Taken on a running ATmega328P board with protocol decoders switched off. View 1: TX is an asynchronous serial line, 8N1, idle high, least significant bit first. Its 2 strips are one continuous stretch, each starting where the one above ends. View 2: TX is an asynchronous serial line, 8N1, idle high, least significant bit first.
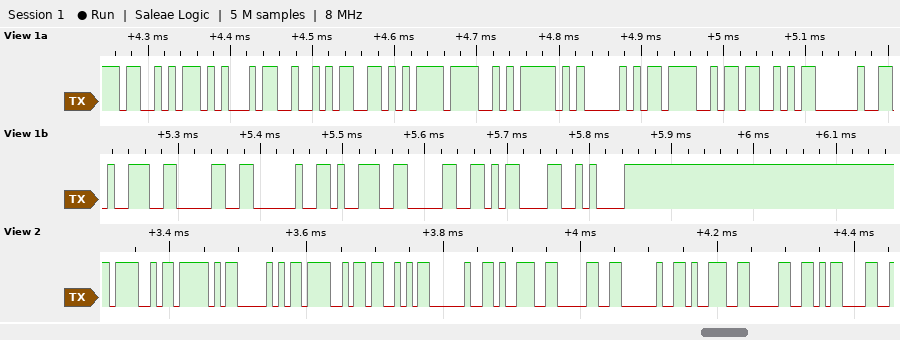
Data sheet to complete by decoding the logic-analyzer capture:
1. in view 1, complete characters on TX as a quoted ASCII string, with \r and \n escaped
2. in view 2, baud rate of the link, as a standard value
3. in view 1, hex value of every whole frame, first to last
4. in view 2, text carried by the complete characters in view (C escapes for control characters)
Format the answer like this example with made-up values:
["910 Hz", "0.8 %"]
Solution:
["\"SERVO_POS 90 90\\r\\n\"", "115200 baud", "0x53 0x45 0x52 0x56 0x4F 0x5F 0x50 0x4F 0x53 0x20 0x39 0x30 0x20 0x39 0x30 0x0D 0x0A", "\"O_POS 90 90\\r\""]
